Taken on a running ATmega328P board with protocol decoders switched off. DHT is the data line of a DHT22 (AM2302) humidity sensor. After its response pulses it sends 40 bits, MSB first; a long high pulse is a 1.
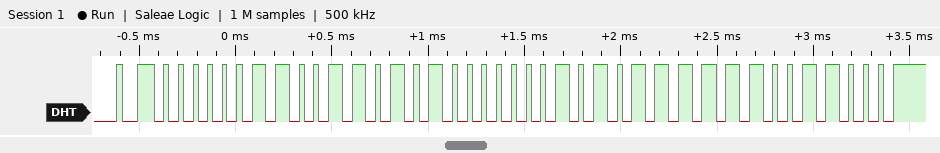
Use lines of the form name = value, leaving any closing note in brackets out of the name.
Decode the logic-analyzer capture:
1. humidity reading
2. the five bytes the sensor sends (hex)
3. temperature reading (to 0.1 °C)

humidity reading = 82.1 %
the five bytes the sensor sends = 03 35 01 5F 98
temperature reading = 35.1 °C
